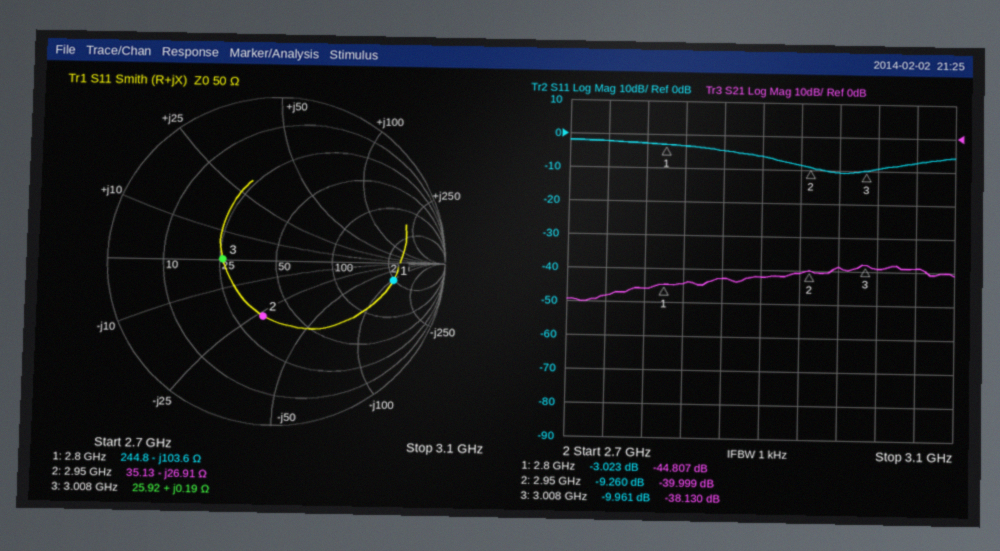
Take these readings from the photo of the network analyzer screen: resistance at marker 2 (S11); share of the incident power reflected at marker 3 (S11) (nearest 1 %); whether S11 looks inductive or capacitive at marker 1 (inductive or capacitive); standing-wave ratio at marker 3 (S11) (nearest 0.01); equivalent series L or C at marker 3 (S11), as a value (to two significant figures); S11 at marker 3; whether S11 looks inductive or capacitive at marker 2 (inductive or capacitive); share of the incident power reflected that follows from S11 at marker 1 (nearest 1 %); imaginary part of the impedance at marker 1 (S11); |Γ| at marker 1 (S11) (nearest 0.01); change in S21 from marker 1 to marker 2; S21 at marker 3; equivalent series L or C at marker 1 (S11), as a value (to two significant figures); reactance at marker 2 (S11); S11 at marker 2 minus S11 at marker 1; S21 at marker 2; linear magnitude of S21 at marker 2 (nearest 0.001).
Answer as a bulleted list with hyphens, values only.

- 35.13 Ω
- 10 %
- capacitive
- 1.93
- 10 pH
- -9.961 dB
- capacitive
- 50 %
- -103.6 Ω
- 0.71
- 4.808 dB
- -38.130 dB
- 550 fF
- -26.91 Ω
- -6.237 dB
- -39.999 dB
- 0.010
